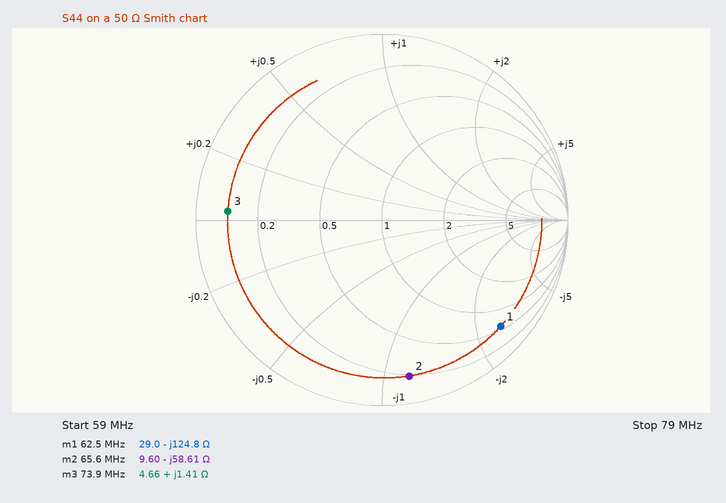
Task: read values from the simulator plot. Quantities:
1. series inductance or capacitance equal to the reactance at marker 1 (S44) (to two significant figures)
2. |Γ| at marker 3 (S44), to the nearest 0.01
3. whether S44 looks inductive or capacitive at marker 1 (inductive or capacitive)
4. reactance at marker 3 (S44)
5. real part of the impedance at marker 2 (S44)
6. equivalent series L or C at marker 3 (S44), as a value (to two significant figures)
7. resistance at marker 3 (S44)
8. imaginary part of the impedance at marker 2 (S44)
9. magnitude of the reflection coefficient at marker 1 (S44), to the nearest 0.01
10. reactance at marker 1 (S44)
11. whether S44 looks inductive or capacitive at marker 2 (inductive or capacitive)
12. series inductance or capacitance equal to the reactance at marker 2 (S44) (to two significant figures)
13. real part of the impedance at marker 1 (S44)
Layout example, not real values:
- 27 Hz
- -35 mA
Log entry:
- 20 pF
- 0.83
- capacitive
- +1.41 Ω
- 9.60 Ω
- 3.0 nH
- 4.66 Ω
- -58.61 Ω
- 0.86
- -124.8 Ω
- capacitive
- 41 pF
- 29.0 Ω
